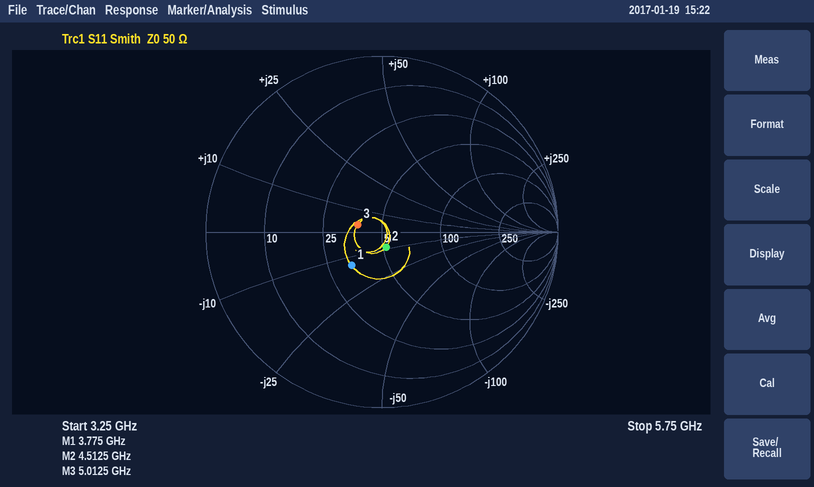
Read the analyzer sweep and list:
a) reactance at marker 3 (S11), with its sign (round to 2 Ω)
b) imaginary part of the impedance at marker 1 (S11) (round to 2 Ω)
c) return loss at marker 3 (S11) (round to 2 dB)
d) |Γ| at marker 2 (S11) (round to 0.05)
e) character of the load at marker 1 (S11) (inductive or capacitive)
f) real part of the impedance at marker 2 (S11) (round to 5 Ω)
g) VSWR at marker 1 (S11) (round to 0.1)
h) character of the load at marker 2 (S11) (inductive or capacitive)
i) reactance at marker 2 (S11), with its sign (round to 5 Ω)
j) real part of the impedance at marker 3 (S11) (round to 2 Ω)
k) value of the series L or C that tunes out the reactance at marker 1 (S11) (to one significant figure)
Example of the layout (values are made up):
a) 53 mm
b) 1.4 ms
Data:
a) +4 Ω
b) -14 Ω
c) 16 dB
d) 0.10
e) capacitive
f) 50 Ω
g) 1.7
h) capacitive
i) -10 Ω
j) 38 Ω
k) 600 pH
